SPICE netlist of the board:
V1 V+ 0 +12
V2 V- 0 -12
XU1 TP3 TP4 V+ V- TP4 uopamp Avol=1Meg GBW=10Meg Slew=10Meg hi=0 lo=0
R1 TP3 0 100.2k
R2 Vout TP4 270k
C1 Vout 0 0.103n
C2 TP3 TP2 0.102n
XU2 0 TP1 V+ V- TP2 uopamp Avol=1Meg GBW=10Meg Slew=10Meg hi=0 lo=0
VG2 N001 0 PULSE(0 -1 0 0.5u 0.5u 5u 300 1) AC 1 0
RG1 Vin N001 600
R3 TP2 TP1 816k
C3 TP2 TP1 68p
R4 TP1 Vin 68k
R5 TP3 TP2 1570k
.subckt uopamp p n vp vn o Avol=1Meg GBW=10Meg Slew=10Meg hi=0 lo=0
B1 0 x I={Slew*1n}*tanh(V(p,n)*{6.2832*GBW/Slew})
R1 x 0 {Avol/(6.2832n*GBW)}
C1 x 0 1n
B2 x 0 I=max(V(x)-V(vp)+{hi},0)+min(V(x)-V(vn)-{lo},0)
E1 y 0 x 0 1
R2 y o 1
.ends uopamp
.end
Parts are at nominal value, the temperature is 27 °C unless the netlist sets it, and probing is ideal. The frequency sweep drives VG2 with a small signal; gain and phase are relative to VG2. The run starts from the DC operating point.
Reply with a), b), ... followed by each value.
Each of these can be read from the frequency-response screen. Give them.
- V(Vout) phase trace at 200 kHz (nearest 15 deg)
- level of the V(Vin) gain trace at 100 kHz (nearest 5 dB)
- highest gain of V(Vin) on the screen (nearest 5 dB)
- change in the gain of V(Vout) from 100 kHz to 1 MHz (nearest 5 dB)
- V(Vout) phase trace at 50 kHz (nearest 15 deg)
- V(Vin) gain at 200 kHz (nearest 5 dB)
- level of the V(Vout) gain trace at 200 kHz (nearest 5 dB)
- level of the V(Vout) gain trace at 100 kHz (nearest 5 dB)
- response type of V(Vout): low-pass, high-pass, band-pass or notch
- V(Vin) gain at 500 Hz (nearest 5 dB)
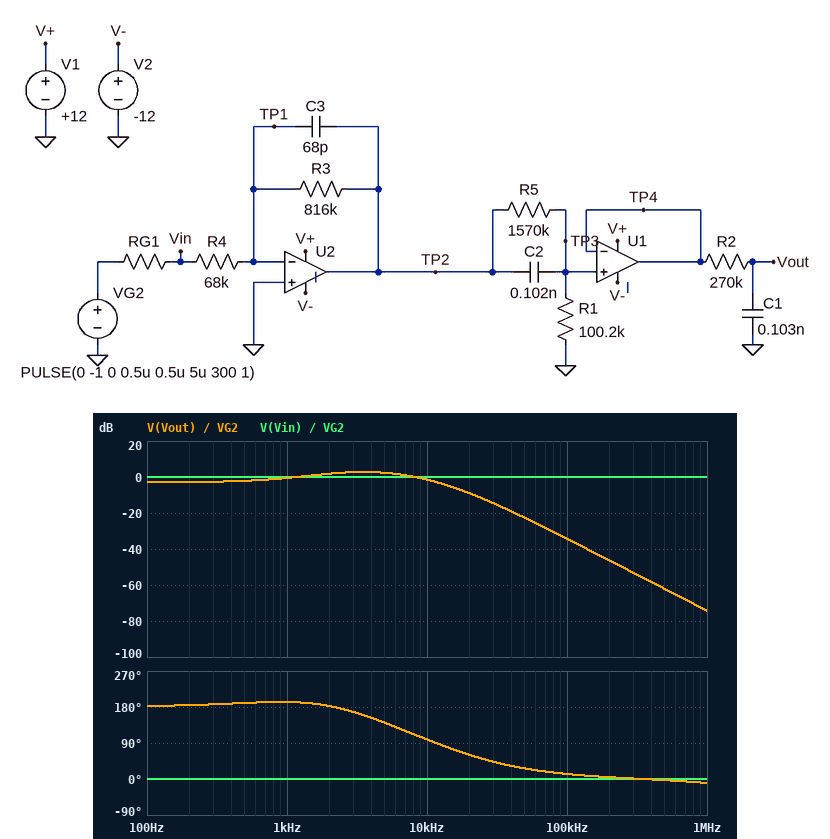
a) 0 deg
b) 0 dB
c) 0 dB
d) -40 dB
e) 30 deg
f) 0 dB
g) -45 dB
h) -35 dB
i) low-pass
j) 0 dB
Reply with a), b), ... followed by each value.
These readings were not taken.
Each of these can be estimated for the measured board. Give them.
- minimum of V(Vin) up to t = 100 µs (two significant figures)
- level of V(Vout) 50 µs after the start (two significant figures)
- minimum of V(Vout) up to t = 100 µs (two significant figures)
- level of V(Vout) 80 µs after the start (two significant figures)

a) -990 mV
b) 47 mV
c) -25 mV
d) -16 mV
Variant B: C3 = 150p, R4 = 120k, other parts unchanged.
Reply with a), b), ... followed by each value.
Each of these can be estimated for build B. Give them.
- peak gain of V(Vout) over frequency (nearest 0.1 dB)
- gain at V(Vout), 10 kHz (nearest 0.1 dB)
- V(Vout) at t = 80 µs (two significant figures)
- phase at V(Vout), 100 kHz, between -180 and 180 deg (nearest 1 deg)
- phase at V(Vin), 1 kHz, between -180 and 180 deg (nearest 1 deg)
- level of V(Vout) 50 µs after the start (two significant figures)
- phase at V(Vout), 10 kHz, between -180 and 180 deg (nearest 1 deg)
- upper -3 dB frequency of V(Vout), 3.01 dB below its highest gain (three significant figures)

a) -6.6 dB
b) -13.0 dB
c) 6.5 mV
d) 12 deg
e) 0 deg
f) 25 mV
g) 90 deg
h) 6.33 kHz
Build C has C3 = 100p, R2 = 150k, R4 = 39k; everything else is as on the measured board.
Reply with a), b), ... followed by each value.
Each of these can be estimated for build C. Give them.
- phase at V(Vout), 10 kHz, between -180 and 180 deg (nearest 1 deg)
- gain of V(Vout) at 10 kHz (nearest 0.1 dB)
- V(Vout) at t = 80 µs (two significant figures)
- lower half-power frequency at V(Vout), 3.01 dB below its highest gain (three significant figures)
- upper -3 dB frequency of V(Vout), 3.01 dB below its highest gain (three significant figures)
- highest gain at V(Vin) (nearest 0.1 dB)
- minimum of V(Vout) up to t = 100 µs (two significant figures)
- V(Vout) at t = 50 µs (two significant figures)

a) 110 deg
b) 3.3 dB
c) -27 mV
d) 749 Hz
e) 10.2 kHz
f) -0.1 dB
g) -30 mV
h) 41 mV
